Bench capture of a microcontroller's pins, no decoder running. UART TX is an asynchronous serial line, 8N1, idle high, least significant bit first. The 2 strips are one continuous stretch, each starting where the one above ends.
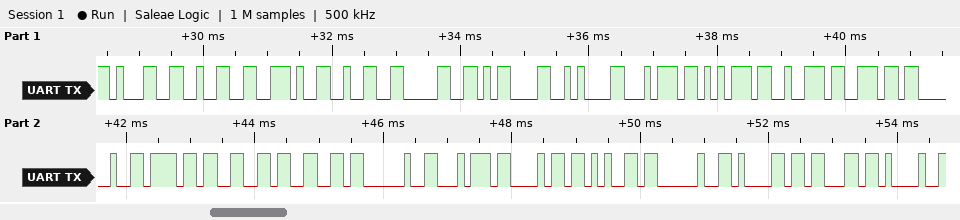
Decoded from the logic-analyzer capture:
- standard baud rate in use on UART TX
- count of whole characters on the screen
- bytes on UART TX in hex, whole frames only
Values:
9600 baud
23
31 32 2E 32 30 0D 0A 74 75 72 6E 20 6F 66 66 20 74 68 65 20 61 63 21
